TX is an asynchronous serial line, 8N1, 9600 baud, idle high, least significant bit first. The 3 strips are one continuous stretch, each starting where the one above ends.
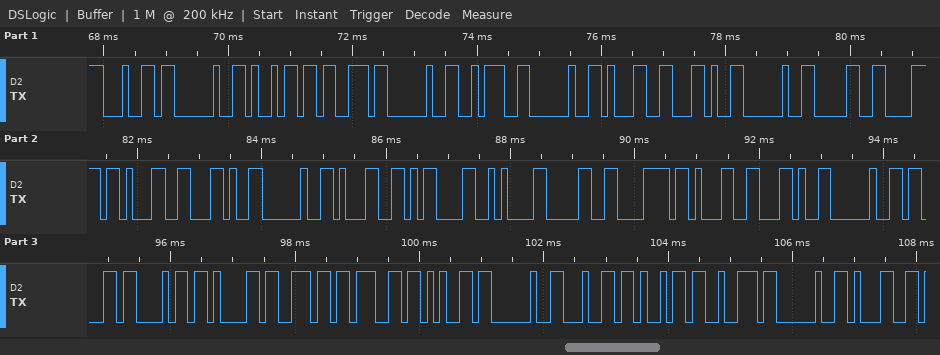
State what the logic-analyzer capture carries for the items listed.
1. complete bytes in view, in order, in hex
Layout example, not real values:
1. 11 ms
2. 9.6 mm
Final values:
1. 64 20 69 73 20 3A 20 31 2C 20 30 78 31 2C 20 31 0D 0A 30 78 31 2C 20 63 68 61 6E 67 65 20 64 69 72 20 31
